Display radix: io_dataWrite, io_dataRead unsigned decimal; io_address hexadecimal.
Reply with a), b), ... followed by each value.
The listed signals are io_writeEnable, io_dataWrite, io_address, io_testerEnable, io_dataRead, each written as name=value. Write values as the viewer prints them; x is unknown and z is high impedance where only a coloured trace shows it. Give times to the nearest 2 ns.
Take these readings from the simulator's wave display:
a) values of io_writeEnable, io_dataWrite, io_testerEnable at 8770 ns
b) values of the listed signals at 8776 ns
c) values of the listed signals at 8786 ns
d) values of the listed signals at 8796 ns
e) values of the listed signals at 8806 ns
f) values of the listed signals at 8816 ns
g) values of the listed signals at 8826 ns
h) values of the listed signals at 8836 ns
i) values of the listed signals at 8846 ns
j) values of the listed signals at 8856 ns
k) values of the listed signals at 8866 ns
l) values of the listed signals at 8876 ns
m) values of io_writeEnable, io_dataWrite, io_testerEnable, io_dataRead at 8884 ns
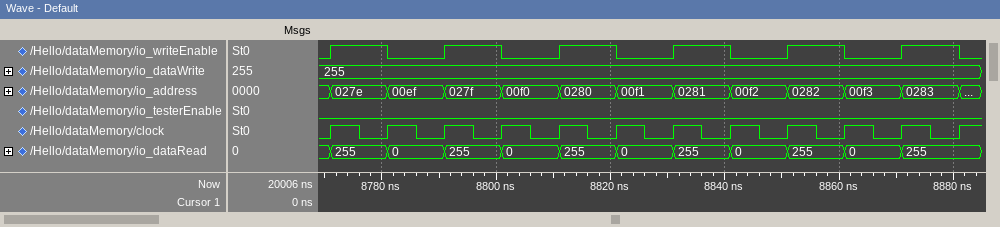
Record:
a) io_writeEnable=0, io_dataWrite=255, io_testerEnable=0
b) io_writeEnable=1, io_dataWrite=255, io_address=027e, io_testerEnable=0, io_dataRead=255
c) io_writeEnable=0, io_dataWrite=255, io_address=00ef, io_testerEnable=0, io_dataRead=0
d) io_writeEnable=1, io_dataWrite=255, io_address=027f, io_testerEnable=0, io_dataRead=255
e) io_writeEnable=0, io_dataWrite=255, io_address=00f0, io_testerEnable=0, io_dataRead=0
f) io_writeEnable=1, io_dataWrite=255, io_address=0280, io_testerEnable=0, io_dataRead=255
g) io_writeEnable=0, io_dataWrite=255, io_address=00f1, io_testerEnable=0, io_dataRead=0
h) io_writeEnable=1, io_dataWrite=255, io_address=0281, io_testerEnable=0, io_dataRead=255
i) io_writeEnable=0, io_dataWrite=255, io_address=00f2, io_testerEnable=0, io_dataRead=0
j) io_writeEnable=1, io_dataWrite=255, io_address=0282, io_testerEnable=0, io_dataRead=255
k) io_writeEnable=0, io_dataWrite=255, io_address=00f3, io_testerEnable=0, io_dataRead=0
l) io_writeEnable=1, io_dataWrite=255, io_address=0283, io_testerEnable=0, io_dataRead=255
m) io_writeEnable=0, io_dataWrite=255, io_testerEnable=0, io_dataRead=255
